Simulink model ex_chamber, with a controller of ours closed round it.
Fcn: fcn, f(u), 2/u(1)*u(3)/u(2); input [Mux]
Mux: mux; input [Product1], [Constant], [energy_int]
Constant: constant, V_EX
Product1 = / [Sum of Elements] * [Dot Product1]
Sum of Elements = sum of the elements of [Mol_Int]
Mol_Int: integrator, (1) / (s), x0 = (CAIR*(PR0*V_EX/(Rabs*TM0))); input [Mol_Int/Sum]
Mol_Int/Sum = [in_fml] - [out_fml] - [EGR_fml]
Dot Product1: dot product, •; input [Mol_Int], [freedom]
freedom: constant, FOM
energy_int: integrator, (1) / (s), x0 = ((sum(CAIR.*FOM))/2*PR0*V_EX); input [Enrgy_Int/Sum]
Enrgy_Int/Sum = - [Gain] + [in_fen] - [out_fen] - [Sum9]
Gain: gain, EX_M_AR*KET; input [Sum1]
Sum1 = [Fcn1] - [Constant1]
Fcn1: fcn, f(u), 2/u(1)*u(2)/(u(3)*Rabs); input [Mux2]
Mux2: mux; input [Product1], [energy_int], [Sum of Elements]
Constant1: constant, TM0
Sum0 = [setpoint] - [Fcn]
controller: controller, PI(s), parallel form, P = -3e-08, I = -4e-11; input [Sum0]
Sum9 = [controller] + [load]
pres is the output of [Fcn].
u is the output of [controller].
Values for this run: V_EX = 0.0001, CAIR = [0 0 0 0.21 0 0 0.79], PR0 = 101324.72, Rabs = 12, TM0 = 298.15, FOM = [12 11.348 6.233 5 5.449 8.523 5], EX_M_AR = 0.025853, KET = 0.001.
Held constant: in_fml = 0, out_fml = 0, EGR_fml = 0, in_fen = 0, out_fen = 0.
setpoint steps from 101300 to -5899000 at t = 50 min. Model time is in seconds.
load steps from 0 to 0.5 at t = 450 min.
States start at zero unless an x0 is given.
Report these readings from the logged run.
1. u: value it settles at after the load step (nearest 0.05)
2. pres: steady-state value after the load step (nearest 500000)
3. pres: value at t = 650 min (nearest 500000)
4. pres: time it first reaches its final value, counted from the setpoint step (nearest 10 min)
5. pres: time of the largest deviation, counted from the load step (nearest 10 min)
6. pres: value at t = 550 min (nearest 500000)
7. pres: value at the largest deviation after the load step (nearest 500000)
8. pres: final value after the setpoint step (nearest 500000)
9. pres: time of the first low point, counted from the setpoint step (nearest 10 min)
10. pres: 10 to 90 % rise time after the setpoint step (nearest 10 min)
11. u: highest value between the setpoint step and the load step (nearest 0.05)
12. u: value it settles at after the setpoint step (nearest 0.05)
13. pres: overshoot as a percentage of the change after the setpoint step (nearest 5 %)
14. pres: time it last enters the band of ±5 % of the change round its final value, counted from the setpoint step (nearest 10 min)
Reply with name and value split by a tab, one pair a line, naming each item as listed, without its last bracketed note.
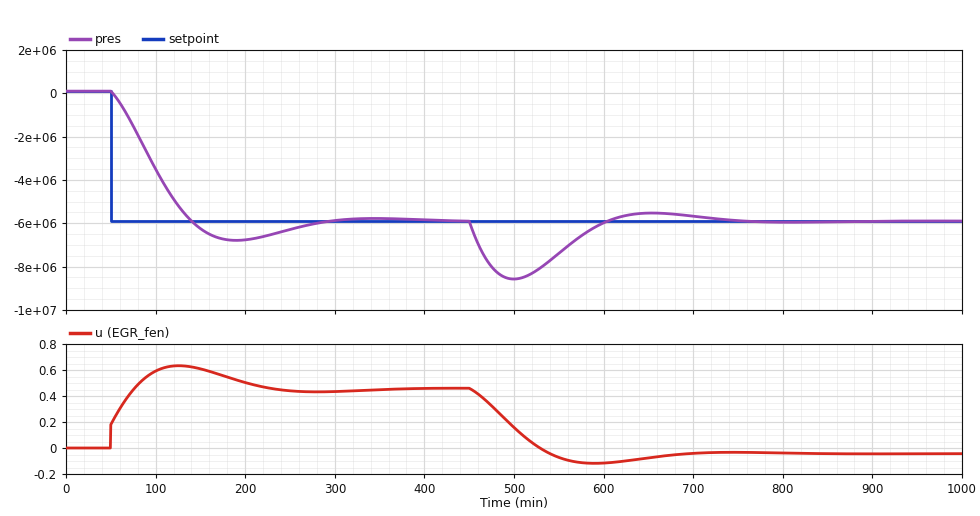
u: value it settles at after the load step	-0.05
pres: steady-state value after the load step	-6000000
pres: value at t = 650 min	-5500000
pres: time it first reaches its final value, counted from the setpoint step	90 min
pres: time of the largest deviation, counted from the load step	50 min
pres: value at t = 550 min	-7500000
pres: value at the largest deviation after the load step	-8500000
pres: final value after the setpoint step	-6000000
pres: time of the first low point, counted from the setpoint step	140 min
pres: 10 to 90 % rise time after the setpoint step	70 min
u: highest value between the setpoint step and the load step	0.65
u: value it settles at after the setpoint step	0.45
pres: overshoot as a percentage of the change after the setpoint step	15 %
pres: time it last enters the band of ±5 % of the change round its final value, counted from the setpoint step	210 min
